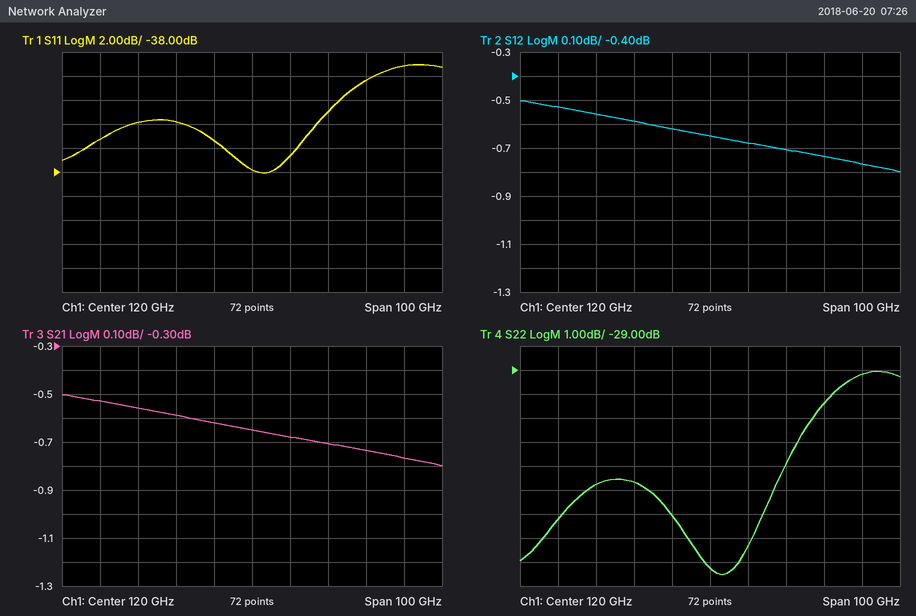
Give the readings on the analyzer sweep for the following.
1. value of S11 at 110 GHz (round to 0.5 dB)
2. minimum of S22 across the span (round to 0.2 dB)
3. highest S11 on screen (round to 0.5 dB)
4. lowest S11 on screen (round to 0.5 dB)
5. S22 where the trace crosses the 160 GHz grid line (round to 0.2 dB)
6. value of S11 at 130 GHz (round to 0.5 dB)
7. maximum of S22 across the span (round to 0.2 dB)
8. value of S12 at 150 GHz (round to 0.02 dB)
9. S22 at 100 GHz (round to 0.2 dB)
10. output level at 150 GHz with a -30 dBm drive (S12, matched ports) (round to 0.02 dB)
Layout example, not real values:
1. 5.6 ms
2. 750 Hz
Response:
1. -35.5 dB
2. -37.6 dB
3. -29.0 dB
4. -38.0 dB
5. -29.2 dB
6. -36.5 dB
7. -29.0 dB
8. -0.74 dB
9. -33.6 dB
10. -30.74 dBm
